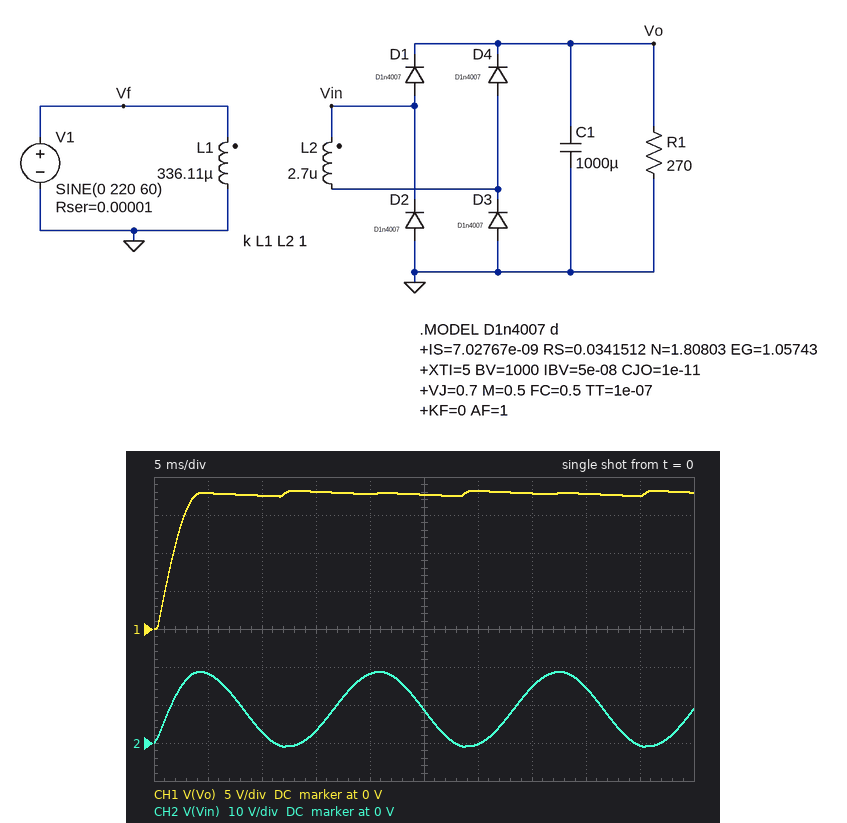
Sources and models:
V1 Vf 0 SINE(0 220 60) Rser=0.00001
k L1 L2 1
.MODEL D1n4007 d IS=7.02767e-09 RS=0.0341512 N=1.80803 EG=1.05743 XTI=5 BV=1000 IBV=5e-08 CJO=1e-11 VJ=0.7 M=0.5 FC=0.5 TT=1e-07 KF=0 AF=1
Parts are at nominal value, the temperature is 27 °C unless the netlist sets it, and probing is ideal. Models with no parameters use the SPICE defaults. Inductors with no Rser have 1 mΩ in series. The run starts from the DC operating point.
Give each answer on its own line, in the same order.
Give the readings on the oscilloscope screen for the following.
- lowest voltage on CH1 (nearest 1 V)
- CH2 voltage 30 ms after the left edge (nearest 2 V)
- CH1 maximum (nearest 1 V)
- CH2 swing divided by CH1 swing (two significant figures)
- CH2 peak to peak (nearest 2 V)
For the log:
0 V
0 V
18 V
1.1
20 V
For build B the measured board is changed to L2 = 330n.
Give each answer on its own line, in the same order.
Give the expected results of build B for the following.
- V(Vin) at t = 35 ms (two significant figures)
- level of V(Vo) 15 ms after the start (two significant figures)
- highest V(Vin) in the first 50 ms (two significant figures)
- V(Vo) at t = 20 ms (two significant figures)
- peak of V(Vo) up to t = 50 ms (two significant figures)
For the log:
4.7 V
5.3 V
6.1 V
5.2 V
5.4 V
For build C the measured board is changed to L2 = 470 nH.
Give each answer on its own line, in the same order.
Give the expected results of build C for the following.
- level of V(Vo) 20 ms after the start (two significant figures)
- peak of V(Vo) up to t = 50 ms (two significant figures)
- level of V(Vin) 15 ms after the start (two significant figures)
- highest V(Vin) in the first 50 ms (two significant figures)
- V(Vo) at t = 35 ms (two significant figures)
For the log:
6.5 V
6.7 V
900 mV
7.4 V
6.6 V
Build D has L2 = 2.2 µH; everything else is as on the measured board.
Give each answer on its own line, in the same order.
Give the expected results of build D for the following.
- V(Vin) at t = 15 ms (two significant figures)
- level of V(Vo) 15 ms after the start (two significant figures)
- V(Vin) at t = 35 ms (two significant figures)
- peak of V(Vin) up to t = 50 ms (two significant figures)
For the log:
2.8 V
16 V
13 V
17 V
